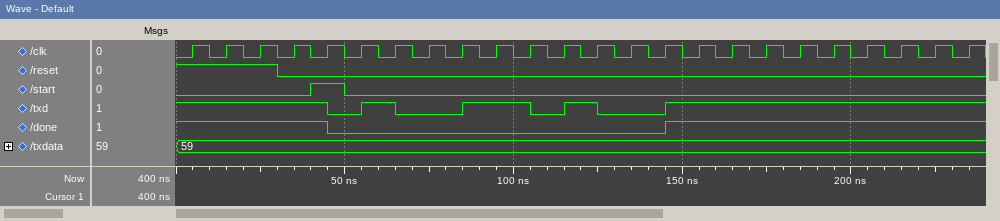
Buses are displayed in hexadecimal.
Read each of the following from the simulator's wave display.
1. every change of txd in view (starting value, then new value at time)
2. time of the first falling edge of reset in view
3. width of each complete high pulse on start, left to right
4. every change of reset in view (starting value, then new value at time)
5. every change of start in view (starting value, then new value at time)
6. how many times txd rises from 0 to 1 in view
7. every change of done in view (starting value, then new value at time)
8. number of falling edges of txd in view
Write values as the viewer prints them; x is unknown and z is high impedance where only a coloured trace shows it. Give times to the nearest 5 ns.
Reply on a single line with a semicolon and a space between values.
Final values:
1, 0 at 45 ns, 1 at 55 ns, 0 at 65 ns, 1 at 85 ns, 0 at 105 ns, 1 at 115 ns, 0 at 125 ns, 1 at 145 ns; 30 ns; 10 ns; 1, 0 at 30 ns; 0, 1 at 40 ns, 0 at 50 ns; 4; 1, 0 at 45 ns, 1 at 145 ns; 4
